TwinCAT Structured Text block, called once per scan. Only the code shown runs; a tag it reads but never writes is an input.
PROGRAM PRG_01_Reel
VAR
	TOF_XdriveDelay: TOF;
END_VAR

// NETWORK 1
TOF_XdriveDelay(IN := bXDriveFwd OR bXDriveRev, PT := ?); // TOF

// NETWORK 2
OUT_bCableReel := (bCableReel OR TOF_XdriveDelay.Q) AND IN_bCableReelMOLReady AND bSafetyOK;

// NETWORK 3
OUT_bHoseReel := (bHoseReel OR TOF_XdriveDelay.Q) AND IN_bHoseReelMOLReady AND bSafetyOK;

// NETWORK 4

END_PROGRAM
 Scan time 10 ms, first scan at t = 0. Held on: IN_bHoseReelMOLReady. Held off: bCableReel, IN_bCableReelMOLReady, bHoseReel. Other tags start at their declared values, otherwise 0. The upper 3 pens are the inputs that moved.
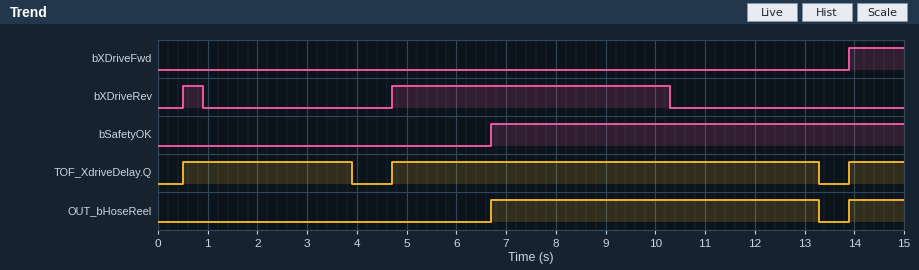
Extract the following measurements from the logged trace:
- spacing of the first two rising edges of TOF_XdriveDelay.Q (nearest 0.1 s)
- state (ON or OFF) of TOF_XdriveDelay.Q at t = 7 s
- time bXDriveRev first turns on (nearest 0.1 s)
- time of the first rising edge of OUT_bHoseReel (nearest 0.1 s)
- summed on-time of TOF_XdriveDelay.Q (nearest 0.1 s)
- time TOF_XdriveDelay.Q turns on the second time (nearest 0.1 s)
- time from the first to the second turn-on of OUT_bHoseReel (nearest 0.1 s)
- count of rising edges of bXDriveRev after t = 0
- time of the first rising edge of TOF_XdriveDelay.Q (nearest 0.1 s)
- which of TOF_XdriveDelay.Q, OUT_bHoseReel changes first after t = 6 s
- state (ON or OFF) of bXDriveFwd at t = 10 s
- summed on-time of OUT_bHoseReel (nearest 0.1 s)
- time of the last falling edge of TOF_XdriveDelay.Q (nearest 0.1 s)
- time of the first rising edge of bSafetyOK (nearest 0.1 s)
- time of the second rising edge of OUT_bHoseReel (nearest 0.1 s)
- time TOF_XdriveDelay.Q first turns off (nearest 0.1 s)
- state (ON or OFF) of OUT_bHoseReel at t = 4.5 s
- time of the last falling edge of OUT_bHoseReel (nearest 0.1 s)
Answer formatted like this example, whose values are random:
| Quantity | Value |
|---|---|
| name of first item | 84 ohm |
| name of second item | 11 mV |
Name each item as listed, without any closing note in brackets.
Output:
| Quantity | Value |
|---|---|
| spacing of the first two rising edges of TOF_XdriveDelay.Q | 4.2 s |
| state (ON or OFF) of TOF_XdriveDelay.Q at t = 7 s | ON |
| time bXDriveRev first turns on | 0.5 s |
| time of the first rising edge of OUT_bHoseReel | 6.7 s |
| summed on-time of TOF_XdriveDelay.Q | 13.1 s |
| time TOF_XdriveDelay.Q turns on the second time | 4.7 s |
| time from the first to the second turn-on of OUT_bHoseReel | 7.2 s |
| count of rising edges of bXDriveRev after t = 0 | 2 |
| time of the first rising edge of TOF_XdriveDelay.Q | 0.5 s |
| which of TOF_XdriveDelay.Q, OUT_bHoseReel changes first after t = 6 s | OUT_bHoseReel |
| state (ON or OFF) of bXDriveFwd at t = 10 s | OFF |
| summed on-time of OUT_bHoseReel | 7.7 s |
| time of the last falling edge of TOF_XdriveDelay.Q | 13.3 s |
| time of the first rising edge of bSafetyOK | 6.7 s |
| time of the second rising edge of OUT_bHoseReel | 13.9 s |
| time TOF_XdriveDelay.Q first turns off | 3.9 s |
| state (ON or OFF) of OUT_bHoseReel at t = 4.5 s | OFF |
| time of the last falling edge of OUT_bHoseReel | 13.3 s |
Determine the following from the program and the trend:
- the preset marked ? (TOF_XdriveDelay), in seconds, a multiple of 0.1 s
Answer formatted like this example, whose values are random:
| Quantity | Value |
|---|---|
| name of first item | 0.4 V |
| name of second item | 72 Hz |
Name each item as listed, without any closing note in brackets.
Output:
| Quantity | Value |
|---|---|
| the preset marked ? (TOF_XdriveDelay), in seconds, a multiple of 0.1 s | 3.0 s |
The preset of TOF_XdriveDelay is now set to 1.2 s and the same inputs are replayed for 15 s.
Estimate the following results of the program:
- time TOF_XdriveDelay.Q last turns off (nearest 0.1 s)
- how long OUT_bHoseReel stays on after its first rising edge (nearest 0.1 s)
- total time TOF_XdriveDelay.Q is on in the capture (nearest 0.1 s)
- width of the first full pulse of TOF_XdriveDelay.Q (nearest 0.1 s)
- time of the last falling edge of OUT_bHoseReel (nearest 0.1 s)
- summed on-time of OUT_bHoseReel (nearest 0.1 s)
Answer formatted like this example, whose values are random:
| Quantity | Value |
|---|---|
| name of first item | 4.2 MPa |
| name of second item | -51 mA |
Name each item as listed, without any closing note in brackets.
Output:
| Quantity | Value |
|---|---|
| time TOF_XdriveDelay.Q last turns off | 11.5 s |
| how long OUT_bHoseReel stays on after its first rising edge | 4.8 s |
| total time TOF_XdriveDelay.Q is on in the capture | 9.5 s |
| width of the first full pulse of TOF_XdriveDelay.Q | 1.6 s |
| time of the last falling edge of OUT_bHoseReel | 11.5 s |
| summed on-time of OUT_bHoseReel | 5.9 s |
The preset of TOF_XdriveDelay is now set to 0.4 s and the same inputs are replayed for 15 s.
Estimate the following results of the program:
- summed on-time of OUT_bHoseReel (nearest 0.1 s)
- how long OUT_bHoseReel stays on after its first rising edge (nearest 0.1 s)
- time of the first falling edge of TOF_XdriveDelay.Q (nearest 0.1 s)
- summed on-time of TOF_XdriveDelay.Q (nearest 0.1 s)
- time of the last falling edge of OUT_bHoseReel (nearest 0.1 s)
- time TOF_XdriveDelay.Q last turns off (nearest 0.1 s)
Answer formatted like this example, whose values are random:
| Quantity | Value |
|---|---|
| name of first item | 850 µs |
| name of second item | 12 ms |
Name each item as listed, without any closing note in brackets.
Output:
| Quantity | Value |
|---|---|
| summed on-time of OUT_bHoseReel | 5.1 s |
| how long OUT_bHoseReel stays on after its first rising edge | 4.0 s |
| time of the first falling edge of TOF_XdriveDelay.Q | 1.3 s |
| summed on-time of TOF_XdriveDelay.Q | 7.9 s |
| time of the last falling edge of OUT_bHoseReel | 10.7 s |
| time TOF_XdriveDelay.Q last turns off | 10.7 s |
